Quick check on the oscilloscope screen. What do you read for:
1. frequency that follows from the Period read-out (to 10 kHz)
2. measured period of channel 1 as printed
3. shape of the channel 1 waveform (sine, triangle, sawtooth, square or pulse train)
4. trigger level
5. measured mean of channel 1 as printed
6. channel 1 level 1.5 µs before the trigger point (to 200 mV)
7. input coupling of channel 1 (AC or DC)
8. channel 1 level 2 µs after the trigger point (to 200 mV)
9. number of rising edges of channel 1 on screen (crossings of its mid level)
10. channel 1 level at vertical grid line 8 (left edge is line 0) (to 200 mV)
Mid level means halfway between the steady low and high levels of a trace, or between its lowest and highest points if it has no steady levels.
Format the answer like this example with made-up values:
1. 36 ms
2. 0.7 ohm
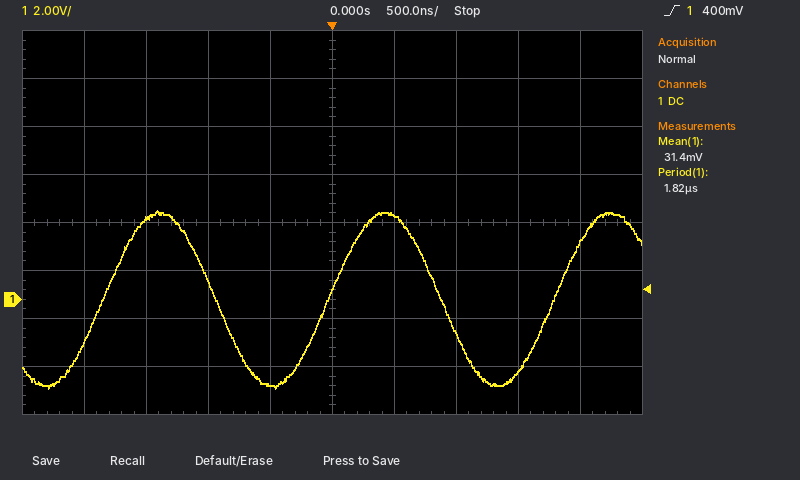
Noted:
1. 550 kHz
2. 1.82 µs
3. sine
4. 400 mV
5. 31.4 mV
6. 3.4 V
7. DC
8. 2.4 V
9. 3
10. -3.0 V
